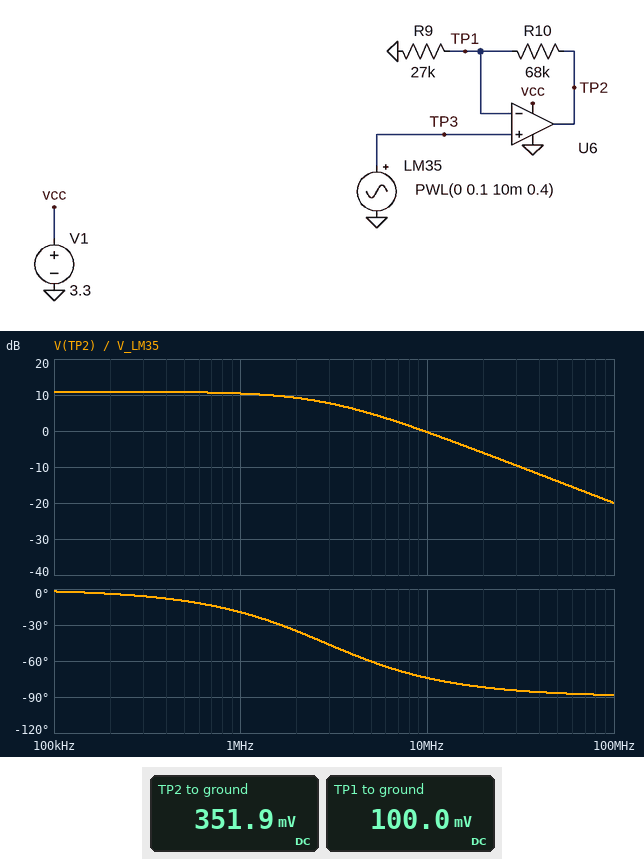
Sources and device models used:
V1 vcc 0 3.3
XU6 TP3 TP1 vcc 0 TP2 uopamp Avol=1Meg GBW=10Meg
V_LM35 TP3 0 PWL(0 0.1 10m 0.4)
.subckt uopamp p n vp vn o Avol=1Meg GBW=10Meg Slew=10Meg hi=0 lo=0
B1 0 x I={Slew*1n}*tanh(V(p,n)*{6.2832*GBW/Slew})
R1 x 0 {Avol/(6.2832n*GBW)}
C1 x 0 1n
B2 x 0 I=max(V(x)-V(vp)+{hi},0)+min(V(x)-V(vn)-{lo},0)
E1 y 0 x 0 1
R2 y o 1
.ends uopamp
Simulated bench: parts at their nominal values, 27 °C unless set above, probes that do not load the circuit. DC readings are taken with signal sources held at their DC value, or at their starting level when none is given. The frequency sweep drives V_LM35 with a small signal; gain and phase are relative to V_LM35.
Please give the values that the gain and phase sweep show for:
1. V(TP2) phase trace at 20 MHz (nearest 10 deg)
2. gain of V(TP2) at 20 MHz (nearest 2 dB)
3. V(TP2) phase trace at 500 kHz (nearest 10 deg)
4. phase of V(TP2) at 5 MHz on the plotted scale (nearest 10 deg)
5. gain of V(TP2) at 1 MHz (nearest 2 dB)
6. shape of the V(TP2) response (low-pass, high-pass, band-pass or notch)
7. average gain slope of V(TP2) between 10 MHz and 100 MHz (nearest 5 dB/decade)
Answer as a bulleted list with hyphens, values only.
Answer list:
- -80 deg
- -6 dB
- -10 deg
- -60 deg
- 10 dB
- low-pass
- -20 dB/decade
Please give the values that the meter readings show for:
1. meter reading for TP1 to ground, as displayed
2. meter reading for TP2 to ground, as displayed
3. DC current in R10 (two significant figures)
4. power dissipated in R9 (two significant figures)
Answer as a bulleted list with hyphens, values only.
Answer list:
- 100.0 mV
- 351.9 mV
- 3.7 µA
- 370 nW
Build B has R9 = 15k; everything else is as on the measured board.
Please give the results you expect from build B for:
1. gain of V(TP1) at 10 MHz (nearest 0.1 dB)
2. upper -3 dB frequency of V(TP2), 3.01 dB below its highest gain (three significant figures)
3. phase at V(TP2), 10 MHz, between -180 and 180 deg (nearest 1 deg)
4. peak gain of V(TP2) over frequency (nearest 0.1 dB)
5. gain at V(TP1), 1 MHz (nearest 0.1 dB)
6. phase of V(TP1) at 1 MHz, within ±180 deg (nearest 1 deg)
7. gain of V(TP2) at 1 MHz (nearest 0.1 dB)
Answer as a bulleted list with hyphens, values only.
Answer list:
- -15.0 dB
- 1.81 MHz
- -80 deg
- 14.9 dB
- -1.2 dB
- -29 deg
- 13.7 dB
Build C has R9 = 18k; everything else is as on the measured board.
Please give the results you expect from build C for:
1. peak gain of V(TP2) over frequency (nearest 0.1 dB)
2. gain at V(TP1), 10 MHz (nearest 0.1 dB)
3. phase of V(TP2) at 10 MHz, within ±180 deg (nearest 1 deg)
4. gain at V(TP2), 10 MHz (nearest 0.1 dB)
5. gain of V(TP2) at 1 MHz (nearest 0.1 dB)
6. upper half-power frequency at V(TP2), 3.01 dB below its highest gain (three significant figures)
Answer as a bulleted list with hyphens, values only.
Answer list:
- 13.6 dB
- -13.8 dB
- -78 deg
- -0.2 dB
- 12.7 dB
- 2.09 MHz
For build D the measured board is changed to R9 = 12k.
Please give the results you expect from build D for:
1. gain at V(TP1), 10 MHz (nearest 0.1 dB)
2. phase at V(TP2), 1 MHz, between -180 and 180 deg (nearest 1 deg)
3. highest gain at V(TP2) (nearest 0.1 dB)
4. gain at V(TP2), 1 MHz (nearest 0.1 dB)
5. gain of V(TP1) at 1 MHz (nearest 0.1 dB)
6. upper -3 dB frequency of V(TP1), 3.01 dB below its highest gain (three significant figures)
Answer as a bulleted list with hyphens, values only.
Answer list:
- -16.6 dB
- -34 deg
- 16.5 dB
- 14.9 dB
- -1.6 dB
- 1.50 MHz
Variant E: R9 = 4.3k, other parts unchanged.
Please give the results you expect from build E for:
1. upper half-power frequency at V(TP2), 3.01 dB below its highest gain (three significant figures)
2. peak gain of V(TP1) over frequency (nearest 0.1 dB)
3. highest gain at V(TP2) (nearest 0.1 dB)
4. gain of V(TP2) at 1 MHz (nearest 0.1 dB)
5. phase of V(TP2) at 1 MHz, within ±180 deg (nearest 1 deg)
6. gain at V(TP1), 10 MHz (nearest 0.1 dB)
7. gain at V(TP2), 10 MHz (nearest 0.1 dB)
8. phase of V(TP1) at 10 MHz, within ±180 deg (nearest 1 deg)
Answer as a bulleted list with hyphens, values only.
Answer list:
- 595 kHz
- 0 dB
- 24.5 dB
- 18.7 dB
- -59 deg
- -24.5 dB
- 0 dB
- -87 deg
